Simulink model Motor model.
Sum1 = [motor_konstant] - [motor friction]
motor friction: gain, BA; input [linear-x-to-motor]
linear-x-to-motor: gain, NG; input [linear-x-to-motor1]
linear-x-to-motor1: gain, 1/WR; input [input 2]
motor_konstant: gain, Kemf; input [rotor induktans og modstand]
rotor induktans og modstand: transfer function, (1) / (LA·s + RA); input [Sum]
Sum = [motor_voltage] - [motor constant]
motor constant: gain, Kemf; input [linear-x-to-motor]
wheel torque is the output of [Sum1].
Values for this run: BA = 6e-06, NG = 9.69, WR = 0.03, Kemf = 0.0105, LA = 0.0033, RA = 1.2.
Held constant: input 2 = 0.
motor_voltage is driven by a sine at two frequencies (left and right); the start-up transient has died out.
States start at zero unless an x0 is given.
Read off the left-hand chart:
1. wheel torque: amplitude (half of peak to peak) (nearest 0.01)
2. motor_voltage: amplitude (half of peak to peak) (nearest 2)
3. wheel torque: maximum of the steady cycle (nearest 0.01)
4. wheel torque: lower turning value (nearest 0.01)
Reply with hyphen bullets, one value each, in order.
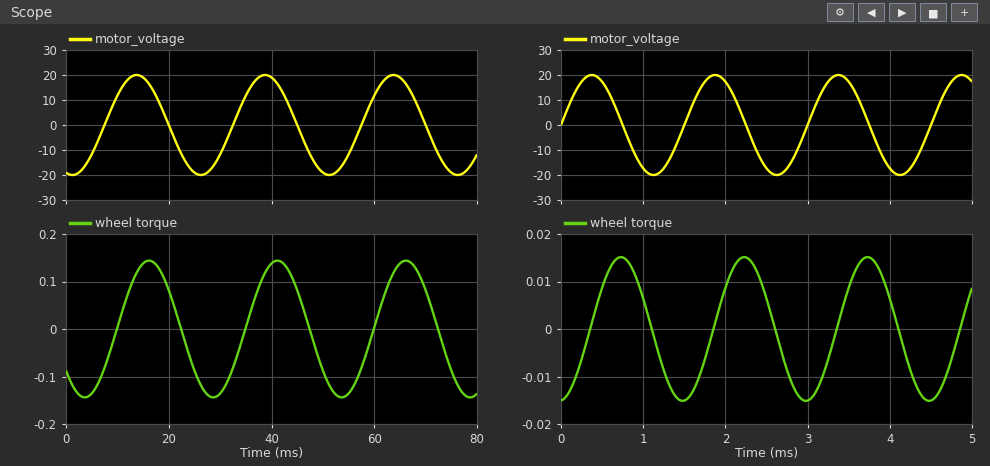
- 0.14
- 20
- 0.14
- -0.14
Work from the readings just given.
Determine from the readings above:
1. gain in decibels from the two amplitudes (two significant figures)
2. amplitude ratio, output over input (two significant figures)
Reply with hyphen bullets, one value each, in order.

- -43 dB
- 0.0070
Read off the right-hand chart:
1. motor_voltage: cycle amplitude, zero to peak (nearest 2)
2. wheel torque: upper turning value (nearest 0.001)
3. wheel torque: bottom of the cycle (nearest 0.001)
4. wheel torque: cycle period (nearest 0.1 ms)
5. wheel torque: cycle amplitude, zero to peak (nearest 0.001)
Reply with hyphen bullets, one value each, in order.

- 20
- 0.015
- -0.015
- 1.5 ms
- 0.015
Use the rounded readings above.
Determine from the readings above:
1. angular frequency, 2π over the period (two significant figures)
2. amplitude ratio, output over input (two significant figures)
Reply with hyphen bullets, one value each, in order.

- 4.2 rad/ms
- 0.00075
